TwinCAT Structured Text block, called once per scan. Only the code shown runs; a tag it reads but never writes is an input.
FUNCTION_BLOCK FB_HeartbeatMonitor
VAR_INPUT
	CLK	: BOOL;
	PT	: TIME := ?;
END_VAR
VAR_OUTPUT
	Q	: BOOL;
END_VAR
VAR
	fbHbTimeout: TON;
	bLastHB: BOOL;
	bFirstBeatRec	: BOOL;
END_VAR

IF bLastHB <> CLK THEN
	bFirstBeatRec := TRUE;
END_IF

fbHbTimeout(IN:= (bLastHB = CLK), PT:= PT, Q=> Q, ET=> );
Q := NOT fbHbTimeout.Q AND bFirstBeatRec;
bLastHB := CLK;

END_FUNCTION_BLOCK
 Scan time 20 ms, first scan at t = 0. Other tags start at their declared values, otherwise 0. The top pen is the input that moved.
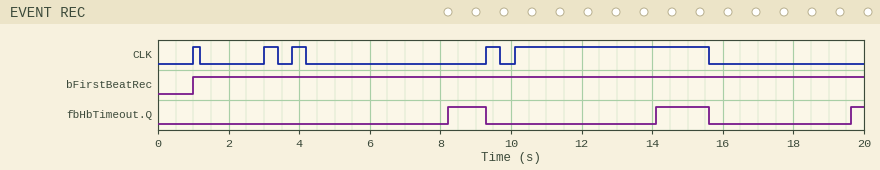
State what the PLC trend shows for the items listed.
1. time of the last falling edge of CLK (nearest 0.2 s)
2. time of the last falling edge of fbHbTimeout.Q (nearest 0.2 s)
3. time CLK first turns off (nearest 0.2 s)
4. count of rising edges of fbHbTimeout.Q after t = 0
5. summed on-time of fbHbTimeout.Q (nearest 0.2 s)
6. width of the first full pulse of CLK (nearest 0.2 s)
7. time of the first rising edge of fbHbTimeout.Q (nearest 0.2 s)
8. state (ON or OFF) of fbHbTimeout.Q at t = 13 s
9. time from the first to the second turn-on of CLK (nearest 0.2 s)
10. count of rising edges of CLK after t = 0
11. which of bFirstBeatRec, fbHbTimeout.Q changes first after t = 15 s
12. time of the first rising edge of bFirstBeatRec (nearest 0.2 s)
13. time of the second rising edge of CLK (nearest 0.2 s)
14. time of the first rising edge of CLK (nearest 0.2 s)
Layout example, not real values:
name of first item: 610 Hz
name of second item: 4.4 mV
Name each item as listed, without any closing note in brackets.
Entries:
time of the last falling edge of CLK: 15.6 s
time of the last falling edge of fbHbTimeout.Q: 15.6 s
time CLK first turns off: 1.2 s
count of rising edges of fbHbTimeout.Q after t = 0: 3
summed on-time of fbHbTimeout.Q: 3.0 s
width of the first full pulse of CLK: 0.2 s
time of the first rising edge of fbHbTimeout.Q: 8.2 s
state (ON or OFF) of fbHbTimeout.Q at t = 13 s: OFF
time from the first to the second turn-on of CLK: 2.0 s
count of rising edges of CLK after t = 0: 5
which of bFirstBeatRec, fbHbTimeout.Q changes first after t = 15 s: fbHbTimeout.Q
time of the first rising edge of bFirstBeatRec: 1.0 s
time of the second rising edge of CLK: 3.0 s
time of the first rising edge of CLK: 1.0 s
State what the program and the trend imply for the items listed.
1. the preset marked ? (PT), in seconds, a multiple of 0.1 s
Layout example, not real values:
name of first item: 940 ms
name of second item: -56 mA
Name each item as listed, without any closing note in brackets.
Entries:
the preset marked ? (PT), in seconds, a multiple of 0.1 s: 4.0 s
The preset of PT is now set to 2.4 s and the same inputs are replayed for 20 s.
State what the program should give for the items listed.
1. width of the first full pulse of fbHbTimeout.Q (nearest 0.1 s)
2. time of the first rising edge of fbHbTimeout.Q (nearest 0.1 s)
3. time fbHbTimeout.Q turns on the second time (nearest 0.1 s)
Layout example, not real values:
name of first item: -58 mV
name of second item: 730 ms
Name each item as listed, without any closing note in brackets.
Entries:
width of the first full pulse of fbHbTimeout.Q: 2.7 s
time of the first rising edge of fbHbTimeout.Q: 6.6 s
time fbHbTimeout.Q turns on the second time: 12.5 s
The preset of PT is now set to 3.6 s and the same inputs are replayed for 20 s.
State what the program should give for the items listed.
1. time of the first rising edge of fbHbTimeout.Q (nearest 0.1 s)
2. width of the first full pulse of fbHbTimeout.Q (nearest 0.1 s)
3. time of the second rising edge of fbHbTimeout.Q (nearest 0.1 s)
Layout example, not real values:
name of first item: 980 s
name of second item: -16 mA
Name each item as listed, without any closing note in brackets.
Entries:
time of the first rising edge of fbHbTimeout.Q: 7.8 s
width of the first full pulse of fbHbTimeout.Q: 1.5 s
time of the second rising edge of fbHbTimeout.Q: 13.7 s
